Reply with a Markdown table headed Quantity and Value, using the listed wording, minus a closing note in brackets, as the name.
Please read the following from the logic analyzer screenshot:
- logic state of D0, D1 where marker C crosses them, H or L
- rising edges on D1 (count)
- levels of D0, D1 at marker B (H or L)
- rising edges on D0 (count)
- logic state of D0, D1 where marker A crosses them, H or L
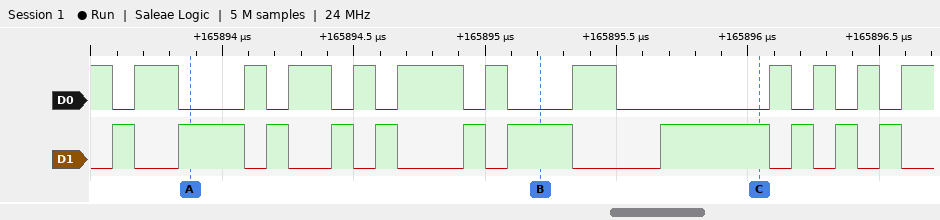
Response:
| Quantity | Value |
|---|---|
| logic state of D0, D1 where marker C crosses them, H or L | D0=L, D1=H |
| rising edges on D1 | 11 |
| levels of D0, D1 at marker B | D0=L, D1=H |
| rising edges on D0 | 11 |
| logic state of D0, D1 where marker A crosses them, H or L | D0=L, D1=H |
